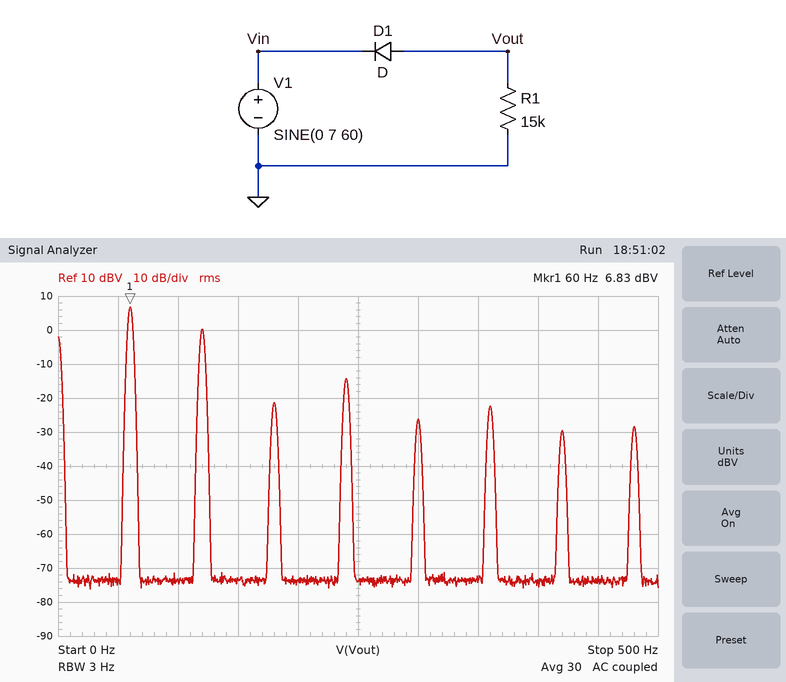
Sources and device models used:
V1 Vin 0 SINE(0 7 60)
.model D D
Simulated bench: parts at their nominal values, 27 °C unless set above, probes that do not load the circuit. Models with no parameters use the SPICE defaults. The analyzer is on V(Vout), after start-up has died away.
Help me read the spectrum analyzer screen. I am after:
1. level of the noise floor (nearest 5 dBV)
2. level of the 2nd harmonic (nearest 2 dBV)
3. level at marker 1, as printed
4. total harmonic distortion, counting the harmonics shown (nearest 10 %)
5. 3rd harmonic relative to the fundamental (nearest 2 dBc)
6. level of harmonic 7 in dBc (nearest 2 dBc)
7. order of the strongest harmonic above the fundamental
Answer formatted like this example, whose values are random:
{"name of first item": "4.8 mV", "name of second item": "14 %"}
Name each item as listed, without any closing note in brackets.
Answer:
{"level of the noise floor": "-75 dBV", "level of the 2nd harmonic": "0 dBV", "level at marker 1, as printed": "6.83 dBV", "total harmonic distortion, counting the harmonics shown": "50 %", "3rd harmonic relative to the fundamental": "-28 dBc", "level of harmonic 7 in dBc": "-36 dBc", "order of the strongest harmonic above the fundamental": "2"}
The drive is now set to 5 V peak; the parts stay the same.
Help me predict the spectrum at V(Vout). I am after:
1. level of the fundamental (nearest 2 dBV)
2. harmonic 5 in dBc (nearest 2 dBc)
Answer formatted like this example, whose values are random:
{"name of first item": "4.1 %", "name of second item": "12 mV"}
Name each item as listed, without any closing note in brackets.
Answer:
{"level of the fundamental": "4 dBV", "harmonic 5 in dBc": "-30 dBc"}
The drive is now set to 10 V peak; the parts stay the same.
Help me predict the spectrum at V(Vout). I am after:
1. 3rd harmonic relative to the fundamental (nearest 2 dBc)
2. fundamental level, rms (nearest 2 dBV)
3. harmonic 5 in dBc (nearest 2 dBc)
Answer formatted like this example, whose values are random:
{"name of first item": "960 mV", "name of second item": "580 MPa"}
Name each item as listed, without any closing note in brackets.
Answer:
{"3rd harmonic relative to the fundamental": "-32 dBc", "fundamental level, rms": "10 dBV", "harmonic 5 in dBc": "-36 dBc"}
